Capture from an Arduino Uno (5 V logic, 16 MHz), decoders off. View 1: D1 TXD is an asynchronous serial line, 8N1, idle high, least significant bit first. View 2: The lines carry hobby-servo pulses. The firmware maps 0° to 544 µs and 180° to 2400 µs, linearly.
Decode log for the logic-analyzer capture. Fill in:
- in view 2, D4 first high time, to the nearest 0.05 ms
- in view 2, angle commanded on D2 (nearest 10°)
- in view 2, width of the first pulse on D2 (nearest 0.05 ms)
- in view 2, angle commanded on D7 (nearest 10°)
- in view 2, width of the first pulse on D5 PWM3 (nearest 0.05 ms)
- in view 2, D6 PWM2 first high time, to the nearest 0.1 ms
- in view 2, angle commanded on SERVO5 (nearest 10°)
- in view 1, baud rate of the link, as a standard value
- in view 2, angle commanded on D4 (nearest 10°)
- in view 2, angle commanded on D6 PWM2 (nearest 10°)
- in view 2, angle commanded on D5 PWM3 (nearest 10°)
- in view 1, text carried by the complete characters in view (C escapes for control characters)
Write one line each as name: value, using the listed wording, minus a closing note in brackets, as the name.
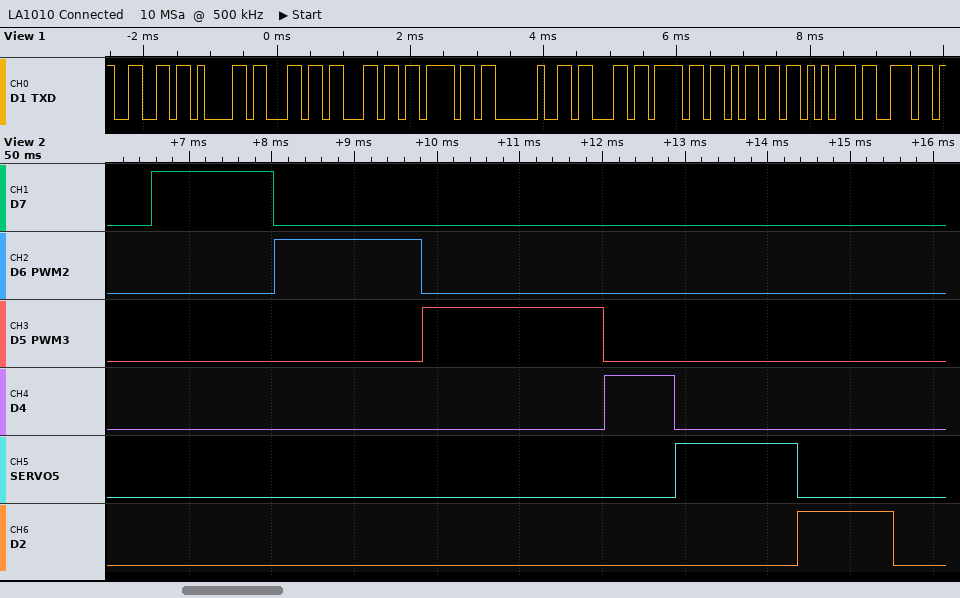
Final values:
in view 2, D4 first high time, to the nearest 0.05 ms: 0.85 ms
in view 2, angle commanded on D2: 60°
in view 2, width of the first pulse on D2: 1.15 ms
in view 2, angle commanded on D7: 90°
in view 2, width of the first pulse on D5 PWM3: 2.20 ms
in view 2, D6 PWM2 first high time, to the nearest 0.1 ms: 1.8 ms
in view 2, angle commanded on SERVO5: 90°
in view 1, baud rate of the link, as a standard value: 9600 baud
in view 2, angle commanded on D4: 30°
in view 2, angle commanded on D6 PWM2: 120°
in view 2, angle commanded on D5 PWM3: 160°
in view 1, text carried by the complete characters in view: "fallo comun"
